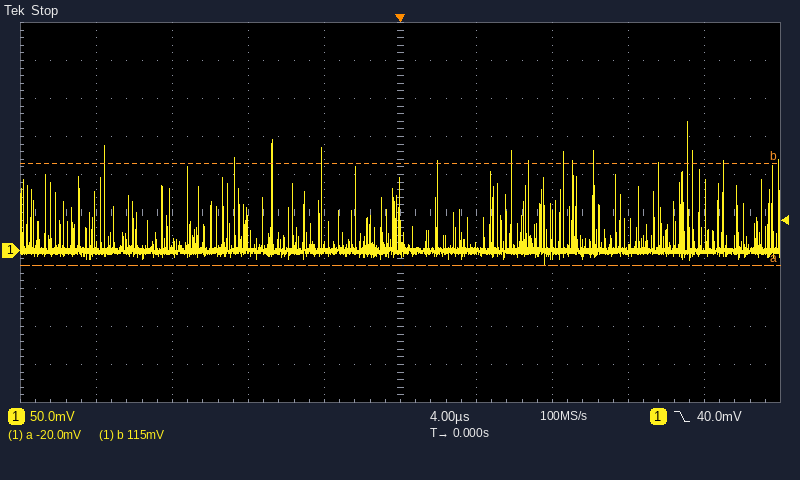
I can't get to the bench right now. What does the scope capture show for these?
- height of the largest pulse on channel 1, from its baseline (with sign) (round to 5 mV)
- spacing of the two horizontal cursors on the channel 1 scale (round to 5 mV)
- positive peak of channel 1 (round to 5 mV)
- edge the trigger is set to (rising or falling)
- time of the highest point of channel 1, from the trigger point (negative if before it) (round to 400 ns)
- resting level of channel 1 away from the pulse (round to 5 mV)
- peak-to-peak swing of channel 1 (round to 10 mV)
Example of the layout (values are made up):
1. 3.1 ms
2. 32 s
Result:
1. +170 mV
2. 135 mV
3. 170 mV
4. falling
5. +15.2 µs
6. 0 mV
7. 190 mV
